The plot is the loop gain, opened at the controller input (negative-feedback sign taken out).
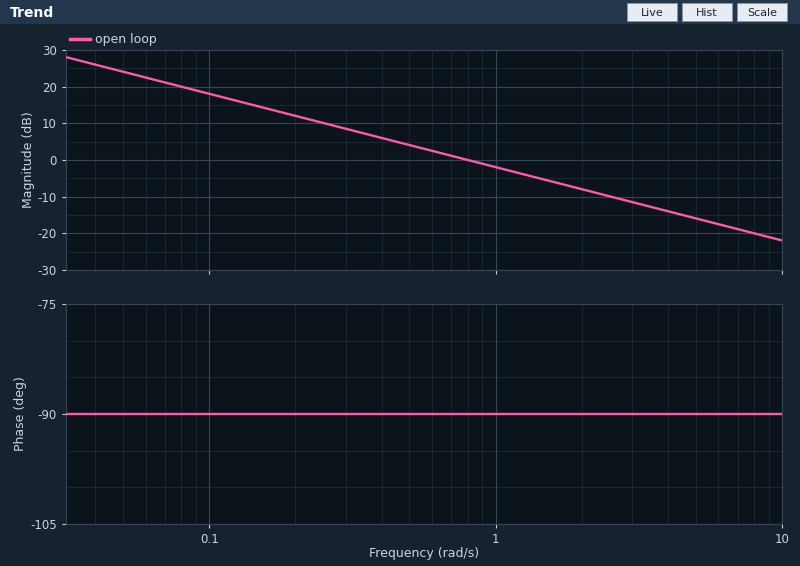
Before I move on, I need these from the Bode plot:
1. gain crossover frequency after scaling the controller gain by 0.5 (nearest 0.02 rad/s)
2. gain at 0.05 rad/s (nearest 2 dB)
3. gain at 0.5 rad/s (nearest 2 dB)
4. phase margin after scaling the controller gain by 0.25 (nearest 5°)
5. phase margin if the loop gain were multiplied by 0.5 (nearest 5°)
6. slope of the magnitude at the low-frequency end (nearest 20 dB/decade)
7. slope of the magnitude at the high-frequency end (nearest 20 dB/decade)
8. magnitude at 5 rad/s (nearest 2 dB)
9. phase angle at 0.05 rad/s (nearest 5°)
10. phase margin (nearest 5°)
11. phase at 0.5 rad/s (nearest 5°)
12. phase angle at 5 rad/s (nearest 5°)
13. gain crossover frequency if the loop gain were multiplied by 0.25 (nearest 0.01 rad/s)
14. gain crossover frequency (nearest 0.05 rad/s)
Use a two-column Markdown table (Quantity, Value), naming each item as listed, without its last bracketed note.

| Quantity | Value |
|---|---|
| gain crossover frequency after scaling the controller gain by 0.5 | 0.40 rad/s |
| gain at 0.05 rad/s | 24 dB |
| gain at 0.5 rad/s | 4 dB |
| phase margin after scaling the controller gain by 0.25 | 90° |
| phase margin if the loop gain were multiplied by 0.5 | 90° |
| slope of the magnitude at the low-frequency end | -20 dB/decade |
| slope of the magnitude at the high-frequency end | -20 dB/decade |
| magnitude at 5 rad/s | -16 dB |
| phase angle at 0.05 rad/s | -90° |
| phase margin | 90° |
| phase at 0.5 rad/s | -90° |
| phase angle at 5 rad/s | -90° |
| gain crossover frequency if the loop gain were multiplied by 0.25 | 0.20 rad/s |
| gain crossover frequency | 0.80 rad/s |
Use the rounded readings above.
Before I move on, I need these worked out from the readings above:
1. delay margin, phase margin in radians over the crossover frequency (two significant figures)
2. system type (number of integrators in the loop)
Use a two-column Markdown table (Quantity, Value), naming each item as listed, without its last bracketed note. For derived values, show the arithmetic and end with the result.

| Quantity | Value |
|---|---|
| delay margin, phase margin in radians over the crossover frequency | 90 × π / 180 / 0.8 = 2.0 s |
| system type | 1 |
